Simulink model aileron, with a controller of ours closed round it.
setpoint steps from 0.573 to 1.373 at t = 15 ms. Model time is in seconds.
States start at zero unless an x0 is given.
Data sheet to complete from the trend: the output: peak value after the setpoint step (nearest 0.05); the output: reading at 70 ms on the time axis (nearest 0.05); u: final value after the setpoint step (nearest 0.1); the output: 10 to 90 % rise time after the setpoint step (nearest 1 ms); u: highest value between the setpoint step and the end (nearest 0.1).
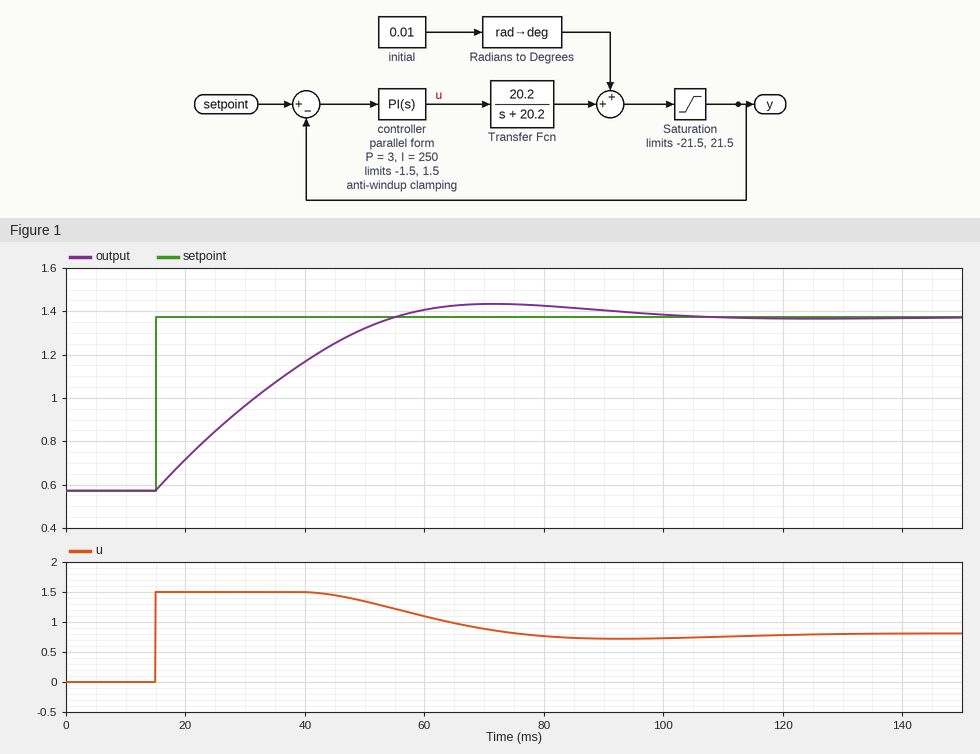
1.45
1.45
0.8
30 ms
1.5
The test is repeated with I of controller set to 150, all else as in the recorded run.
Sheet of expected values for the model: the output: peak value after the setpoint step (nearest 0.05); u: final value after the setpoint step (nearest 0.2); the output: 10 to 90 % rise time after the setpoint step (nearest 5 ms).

1.40
0.8
35 ms
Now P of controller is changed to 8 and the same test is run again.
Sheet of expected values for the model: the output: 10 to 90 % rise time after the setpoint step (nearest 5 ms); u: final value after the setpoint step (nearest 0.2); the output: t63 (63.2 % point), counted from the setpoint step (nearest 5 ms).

35 ms
0.8
20 ms
